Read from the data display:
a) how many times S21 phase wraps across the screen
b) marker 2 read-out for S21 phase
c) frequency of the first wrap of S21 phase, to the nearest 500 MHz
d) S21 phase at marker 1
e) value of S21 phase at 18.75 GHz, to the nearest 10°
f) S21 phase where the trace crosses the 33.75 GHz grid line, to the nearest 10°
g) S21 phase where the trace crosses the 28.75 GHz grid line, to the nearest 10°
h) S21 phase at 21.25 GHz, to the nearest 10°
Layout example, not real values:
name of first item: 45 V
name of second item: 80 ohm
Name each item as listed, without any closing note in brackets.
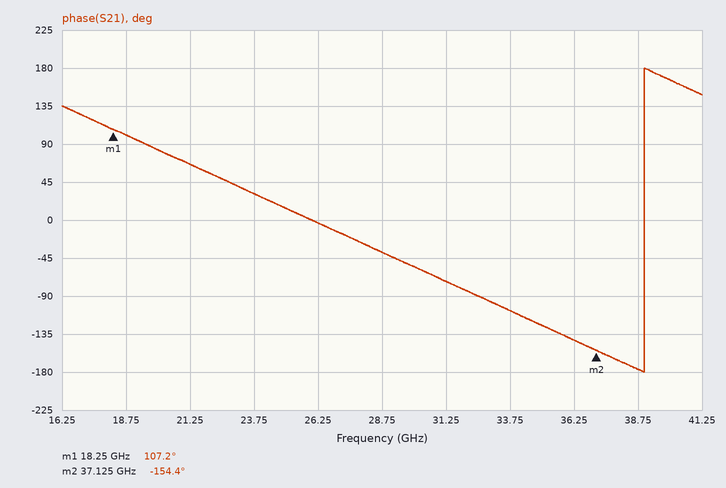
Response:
how many times S21 phase wraps across the screen: 1
marker 2 read-out for S21 phase: -154.4°
frequency of the first wrap of S21 phase, to the nearest 500 MHz: 39.0 GHz
S21 phase at marker 1: 107.2°
value of S21 phase at 18.75 GHz, to the nearest 10°: 100°
S21 phase where the trace crosses the 33.75 GHz grid line, to the nearest 10°: -110°
S21 phase where the trace crosses the 28.75 GHz grid line, to the nearest 10°: -40°
S21 phase at 21.25 GHz, to the nearest 10°: 70°
